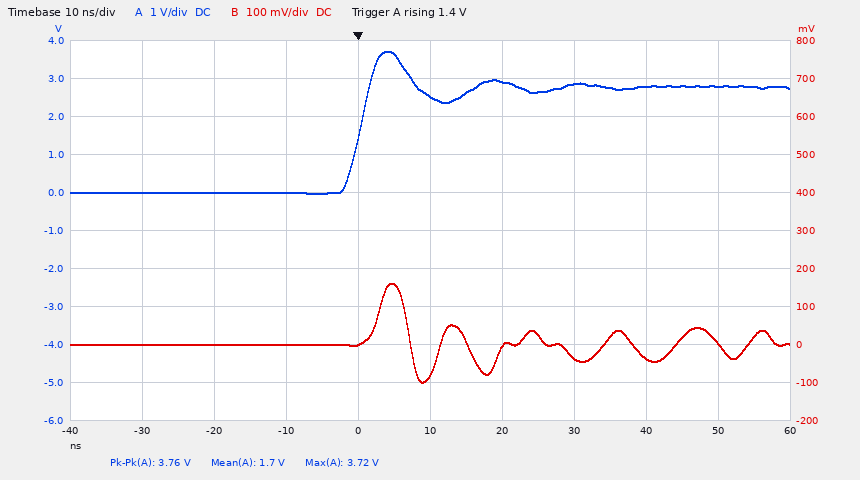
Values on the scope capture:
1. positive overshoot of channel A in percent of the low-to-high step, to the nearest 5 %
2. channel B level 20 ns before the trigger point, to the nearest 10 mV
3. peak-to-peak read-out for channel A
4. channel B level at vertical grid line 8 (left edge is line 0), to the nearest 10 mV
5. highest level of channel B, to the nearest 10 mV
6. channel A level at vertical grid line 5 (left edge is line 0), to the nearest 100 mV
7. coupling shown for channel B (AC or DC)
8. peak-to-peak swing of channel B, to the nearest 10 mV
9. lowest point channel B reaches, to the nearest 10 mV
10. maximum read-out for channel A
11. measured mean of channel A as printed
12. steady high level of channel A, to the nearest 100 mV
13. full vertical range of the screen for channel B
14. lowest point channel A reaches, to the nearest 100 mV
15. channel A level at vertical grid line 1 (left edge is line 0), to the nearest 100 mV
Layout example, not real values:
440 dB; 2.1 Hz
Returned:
35 %; 0 mV; 3.76 V; -40 mV; 160 mV; 2.5 V; DC; 260 mV; -100 mV; 3.72 V; 1.7 V; 2.8 V; 1 V; 0.0 V; 0.0 V
